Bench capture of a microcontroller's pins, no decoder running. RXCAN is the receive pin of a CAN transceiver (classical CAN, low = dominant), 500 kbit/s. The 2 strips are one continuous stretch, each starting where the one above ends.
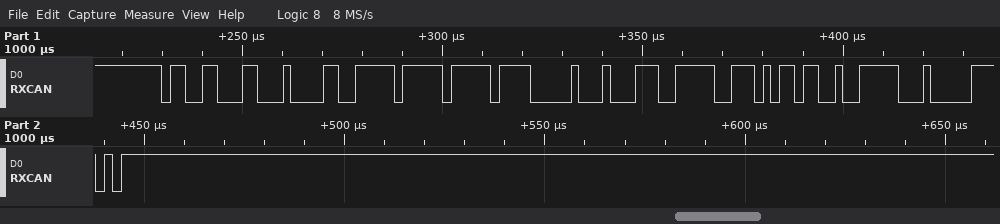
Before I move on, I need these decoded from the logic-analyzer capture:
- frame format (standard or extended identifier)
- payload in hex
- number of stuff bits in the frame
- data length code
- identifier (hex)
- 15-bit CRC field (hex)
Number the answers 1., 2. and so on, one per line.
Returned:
1. standard
2. 67 FF FF 00 8E 7D D6 C9
3. 7
4. 8
5. 0x663
6. 0x7906
